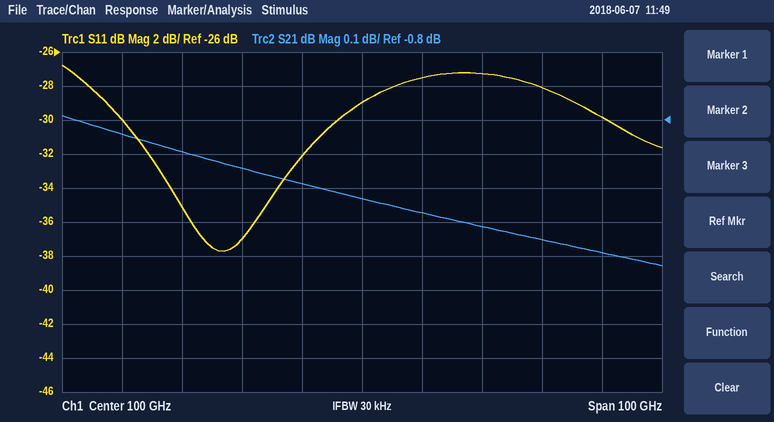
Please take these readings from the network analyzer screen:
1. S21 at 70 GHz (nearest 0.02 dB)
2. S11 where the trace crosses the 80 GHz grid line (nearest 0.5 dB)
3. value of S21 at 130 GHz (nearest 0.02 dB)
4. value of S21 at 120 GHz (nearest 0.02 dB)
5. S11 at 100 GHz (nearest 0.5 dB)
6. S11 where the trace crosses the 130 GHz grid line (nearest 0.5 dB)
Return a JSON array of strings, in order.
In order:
["-0.90 dB", "-37.0 dB", "-1.16 dB", "-1.12 dB", "-29.0 dB", "-28.0 dB"]
